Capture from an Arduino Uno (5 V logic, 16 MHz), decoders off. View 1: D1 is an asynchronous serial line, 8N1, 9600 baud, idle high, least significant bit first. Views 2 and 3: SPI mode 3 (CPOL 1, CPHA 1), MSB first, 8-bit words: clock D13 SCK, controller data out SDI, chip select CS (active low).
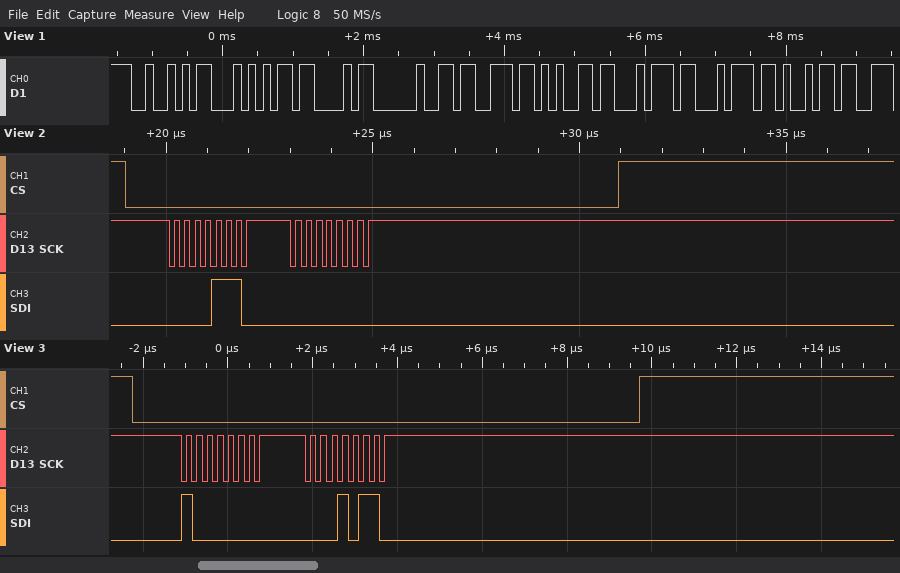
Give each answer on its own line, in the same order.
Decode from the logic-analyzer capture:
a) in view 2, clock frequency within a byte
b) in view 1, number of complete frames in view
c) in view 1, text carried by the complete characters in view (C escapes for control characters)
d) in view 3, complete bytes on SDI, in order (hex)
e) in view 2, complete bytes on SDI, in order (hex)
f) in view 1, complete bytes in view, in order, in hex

4 MHz
9
"RTC setti"
80 16
0E 00
0x52 0x54 0x43 0x20 0x73 0x65 0x74 0x74 0x69
